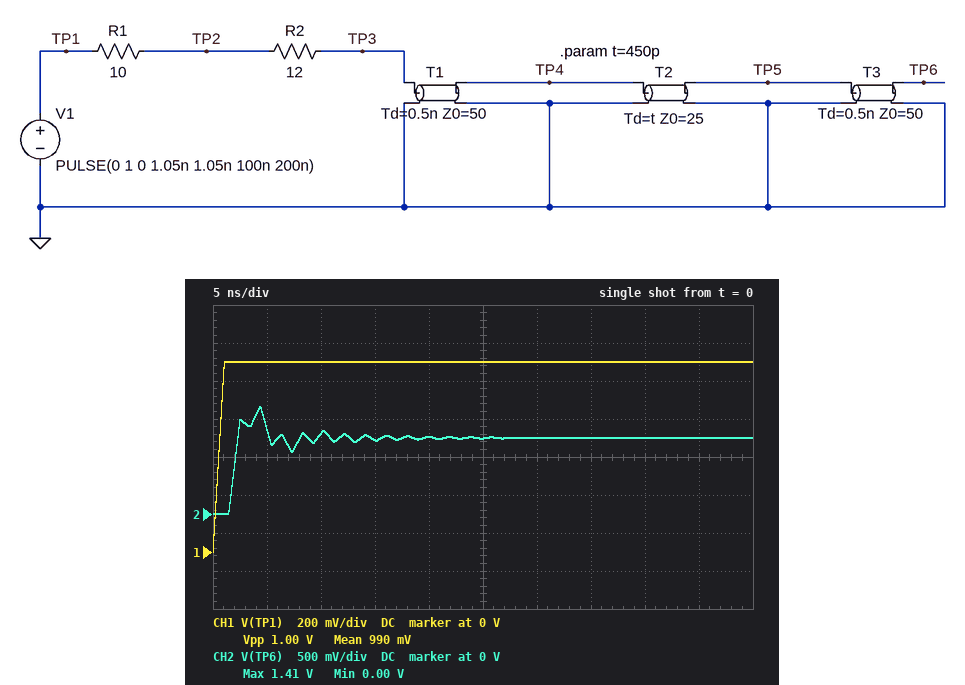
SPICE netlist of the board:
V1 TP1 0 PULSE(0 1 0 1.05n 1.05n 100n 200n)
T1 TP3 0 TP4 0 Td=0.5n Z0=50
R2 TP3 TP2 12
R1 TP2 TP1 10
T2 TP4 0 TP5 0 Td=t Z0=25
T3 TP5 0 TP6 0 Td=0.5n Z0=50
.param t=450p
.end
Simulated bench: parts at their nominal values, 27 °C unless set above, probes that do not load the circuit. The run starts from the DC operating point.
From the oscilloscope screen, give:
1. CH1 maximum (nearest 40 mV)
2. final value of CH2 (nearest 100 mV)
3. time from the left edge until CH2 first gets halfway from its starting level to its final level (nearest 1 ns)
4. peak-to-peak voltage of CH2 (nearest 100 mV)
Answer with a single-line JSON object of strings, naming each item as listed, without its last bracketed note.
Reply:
{"CH1 maximum": "1.00 V", "final value of CH2": "1.0 V", "time from the left edge until CH2 first gets halfway from its starting level to its final level": "2 ns", "peak-to-peak voltage of CH2": "1.4 V"}
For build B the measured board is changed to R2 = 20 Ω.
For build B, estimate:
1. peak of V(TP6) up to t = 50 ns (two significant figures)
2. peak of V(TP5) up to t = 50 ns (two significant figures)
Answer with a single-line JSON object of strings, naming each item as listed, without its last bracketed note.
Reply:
{"peak of V(TP6) up to t = 50 ns": "1.3 V", "peak of V(TP5) up to t = 50 ns": "1.1 V"}
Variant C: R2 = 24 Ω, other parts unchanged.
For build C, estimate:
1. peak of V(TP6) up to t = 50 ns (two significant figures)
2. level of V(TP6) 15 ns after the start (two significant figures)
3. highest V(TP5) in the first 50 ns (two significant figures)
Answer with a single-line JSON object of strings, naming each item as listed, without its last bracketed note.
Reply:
{"peak of V(TP6) up to t = 50 ns": "1.2 V", "level of V(TP6) 15 ns after the start": "990 mV", "highest V(TP5) in the first 50 ns": "1.1 V"}
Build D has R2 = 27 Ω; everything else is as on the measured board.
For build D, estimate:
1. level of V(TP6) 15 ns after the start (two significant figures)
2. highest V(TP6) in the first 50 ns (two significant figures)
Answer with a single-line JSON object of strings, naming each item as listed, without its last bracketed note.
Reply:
{"level of V(TP6) 15 ns after the start": "990 mV", "highest V(TP6) in the first 50 ns": "1.2 V"}
